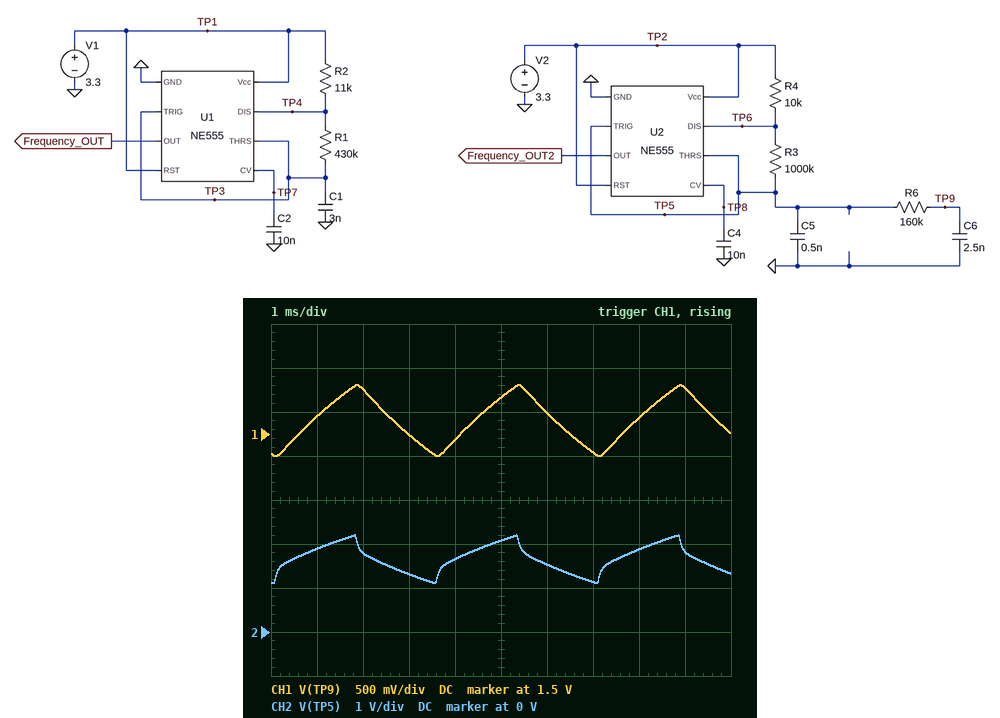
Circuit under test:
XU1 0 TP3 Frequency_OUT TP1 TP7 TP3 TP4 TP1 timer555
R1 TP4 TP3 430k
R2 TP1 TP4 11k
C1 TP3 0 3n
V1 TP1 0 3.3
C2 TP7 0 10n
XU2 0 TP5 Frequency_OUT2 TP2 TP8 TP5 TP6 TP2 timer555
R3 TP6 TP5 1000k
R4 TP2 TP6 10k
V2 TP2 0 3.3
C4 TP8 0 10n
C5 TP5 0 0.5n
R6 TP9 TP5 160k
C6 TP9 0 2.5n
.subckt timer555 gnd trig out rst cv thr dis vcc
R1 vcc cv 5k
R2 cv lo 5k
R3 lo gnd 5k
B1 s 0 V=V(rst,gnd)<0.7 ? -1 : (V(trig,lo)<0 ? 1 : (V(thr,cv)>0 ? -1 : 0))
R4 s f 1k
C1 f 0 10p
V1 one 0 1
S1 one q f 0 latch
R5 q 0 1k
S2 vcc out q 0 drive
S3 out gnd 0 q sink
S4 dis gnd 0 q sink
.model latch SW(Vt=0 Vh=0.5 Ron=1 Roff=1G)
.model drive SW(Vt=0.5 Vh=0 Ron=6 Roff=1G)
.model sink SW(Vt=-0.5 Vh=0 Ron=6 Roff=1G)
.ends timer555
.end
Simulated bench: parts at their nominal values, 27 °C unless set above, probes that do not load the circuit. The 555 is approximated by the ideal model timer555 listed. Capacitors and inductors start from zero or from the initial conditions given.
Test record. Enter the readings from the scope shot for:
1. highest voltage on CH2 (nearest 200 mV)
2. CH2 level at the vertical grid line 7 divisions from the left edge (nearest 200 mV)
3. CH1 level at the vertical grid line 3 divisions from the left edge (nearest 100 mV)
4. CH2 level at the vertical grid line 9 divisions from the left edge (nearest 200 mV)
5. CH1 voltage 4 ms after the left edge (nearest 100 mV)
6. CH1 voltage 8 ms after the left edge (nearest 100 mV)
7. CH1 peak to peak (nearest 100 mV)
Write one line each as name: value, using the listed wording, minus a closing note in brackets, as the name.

highest voltage on CH2: 2.2 V
CH2 level at the vertical grid line 7 divisions from the left edge: 1.2 V
CH1 level at the vertical grid line 3 divisions from the left edge: 1.5 V
CH2 level at the vertical grid line 9 divisions from the left edge: 1.8 V
CH1 voltage 4 ms after the left edge: 1.4 V
CH1 voltage 8 ms after the left edge: 1.7 V
CH1 peak to peak: 800 mV
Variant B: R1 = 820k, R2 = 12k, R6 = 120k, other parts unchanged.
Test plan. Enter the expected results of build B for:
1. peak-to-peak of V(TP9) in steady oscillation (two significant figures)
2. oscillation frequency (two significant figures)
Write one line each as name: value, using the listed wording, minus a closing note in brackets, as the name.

peak-to-peak of V(TP9) in steady oscillation: 890 mV
oscillation frequency: 270 Hz
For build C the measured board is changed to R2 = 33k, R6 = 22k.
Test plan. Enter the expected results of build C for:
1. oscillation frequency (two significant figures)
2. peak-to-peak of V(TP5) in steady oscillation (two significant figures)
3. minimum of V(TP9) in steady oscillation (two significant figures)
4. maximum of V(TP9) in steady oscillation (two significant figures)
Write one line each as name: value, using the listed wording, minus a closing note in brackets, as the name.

oscillation frequency: 240 Hz
peak-to-peak of V(TP5) in steady oscillation: 1.1 V
minimum of V(TP9) in steady oscillation: 1.1 V
maximum of V(TP9) in steady oscillation: 2.2 V
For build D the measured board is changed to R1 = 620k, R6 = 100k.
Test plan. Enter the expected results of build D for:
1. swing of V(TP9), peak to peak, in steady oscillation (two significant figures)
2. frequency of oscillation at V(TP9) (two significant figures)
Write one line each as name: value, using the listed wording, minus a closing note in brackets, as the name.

swing of V(TP9), peak to peak, in steady oscillation: 920 mV
frequency of oscillation at V(TP9): 260 Hz
